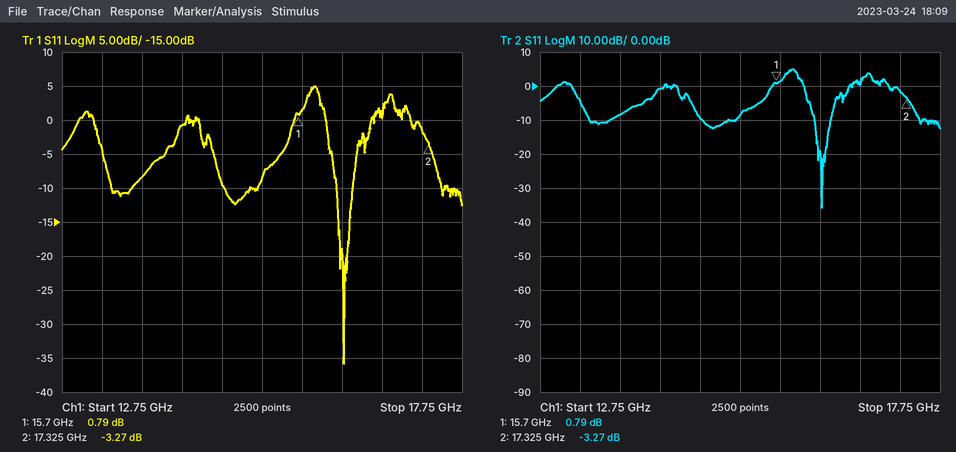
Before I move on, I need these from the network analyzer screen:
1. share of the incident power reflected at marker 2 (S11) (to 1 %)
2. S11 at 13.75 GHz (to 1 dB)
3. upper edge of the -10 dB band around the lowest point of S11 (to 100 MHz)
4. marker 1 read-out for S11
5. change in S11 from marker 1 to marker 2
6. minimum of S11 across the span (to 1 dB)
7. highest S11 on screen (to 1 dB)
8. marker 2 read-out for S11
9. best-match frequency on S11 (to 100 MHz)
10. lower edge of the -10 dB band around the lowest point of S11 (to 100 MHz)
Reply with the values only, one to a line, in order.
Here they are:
47 %
-8 dB
16.4 GHz
0.79 dB
-4.06 dB
-36 dB
5 dB
-3.27 dB
16.3 GHz
16.2 GHz
